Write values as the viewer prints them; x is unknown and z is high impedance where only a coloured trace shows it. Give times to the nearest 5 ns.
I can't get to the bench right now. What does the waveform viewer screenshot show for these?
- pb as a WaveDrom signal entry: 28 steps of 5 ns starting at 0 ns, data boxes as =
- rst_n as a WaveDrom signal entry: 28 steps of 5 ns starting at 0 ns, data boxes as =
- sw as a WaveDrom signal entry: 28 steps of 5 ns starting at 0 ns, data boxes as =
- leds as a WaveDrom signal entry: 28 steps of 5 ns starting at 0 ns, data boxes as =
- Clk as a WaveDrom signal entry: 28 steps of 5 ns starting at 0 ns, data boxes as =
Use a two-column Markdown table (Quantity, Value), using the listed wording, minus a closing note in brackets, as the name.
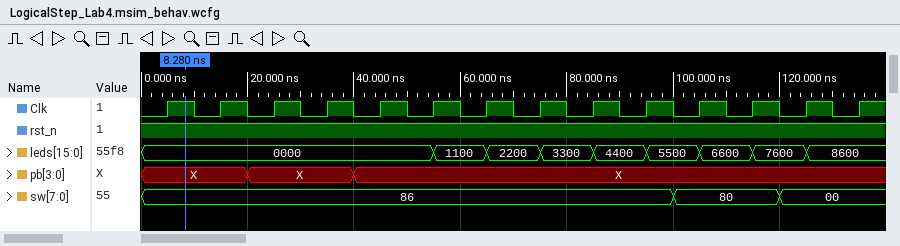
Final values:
| Quantity | Value |
|---|---|
| pb as a WaveDrom signal entry: 28 steps of 5 ns starting at 0 ns, data boxes as = | {name: 'pb', wave: '=...=...=...................', data: 'X X X'} |
| rst_n as a WaveDrom signal entry: 28 steps of 5 ns starting at 0 ns, data boxes as = | {name: 'rst_n', wave: '1...........................'} |
| sw as a WaveDrom signal entry: 28 steps of 5 ns starting at 0 ns, data boxes as = | {name: 'sw', wave: '=...................=...=...', data: '86 80 00'} |
| leds as a WaveDrom signal entry: 28 steps of 5 ns starting at 0 ns, data boxes as = | {name: 'leds', wave: '=..........=.=.=.=.=.=.=.=..', data: '0000 1100 2200 3300 4400 5500 6600 7600 8600'} |
| Clk as a WaveDrom signal entry: 28 steps of 5 ns starting at 0 ns, data boxes as = | {name: 'Clk', wave: '0101010101010101010101010101'} |
